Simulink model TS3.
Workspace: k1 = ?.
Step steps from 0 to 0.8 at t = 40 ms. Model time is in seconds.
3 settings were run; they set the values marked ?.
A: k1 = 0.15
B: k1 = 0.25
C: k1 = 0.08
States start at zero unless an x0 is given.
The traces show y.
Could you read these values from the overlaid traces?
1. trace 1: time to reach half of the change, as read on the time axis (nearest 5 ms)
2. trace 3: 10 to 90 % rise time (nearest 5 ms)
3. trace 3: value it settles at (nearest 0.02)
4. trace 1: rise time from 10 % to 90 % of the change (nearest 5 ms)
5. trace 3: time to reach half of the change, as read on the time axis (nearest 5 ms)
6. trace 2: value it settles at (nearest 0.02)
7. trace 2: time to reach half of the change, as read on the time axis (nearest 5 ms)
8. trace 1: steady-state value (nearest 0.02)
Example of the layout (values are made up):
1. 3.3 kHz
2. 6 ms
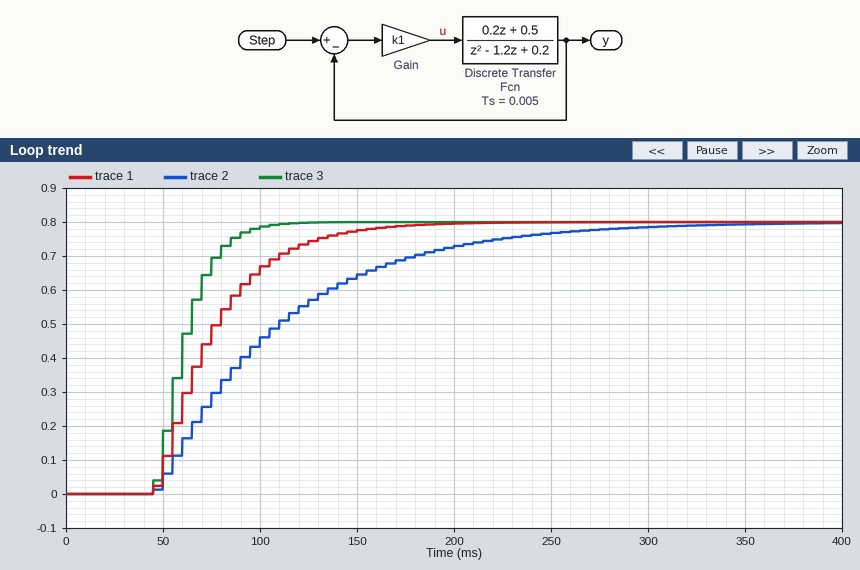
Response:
1. 70 ms
2. 30 ms
3. 0.80
4. 65 ms
5. 60 ms
6. 0.80
7. 90 ms
8. 0.80
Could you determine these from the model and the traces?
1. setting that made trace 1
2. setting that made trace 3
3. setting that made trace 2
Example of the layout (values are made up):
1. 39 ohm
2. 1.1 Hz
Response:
1. A
2. B
3. C
